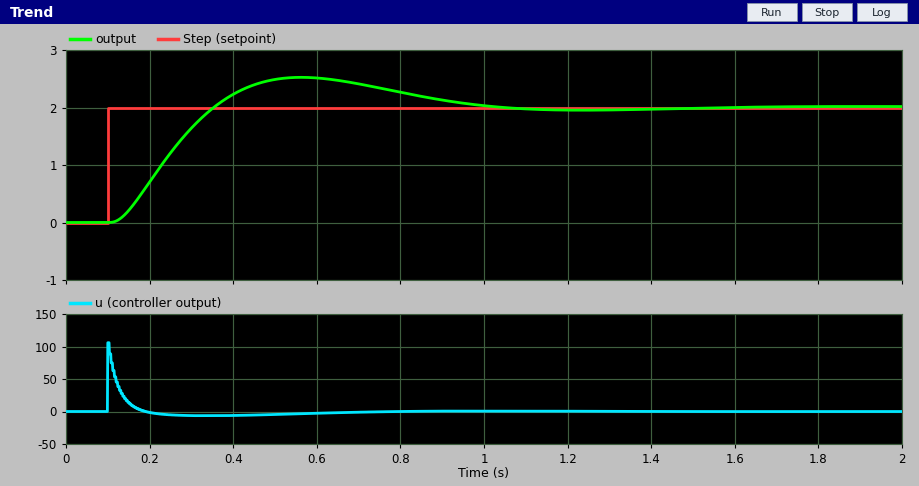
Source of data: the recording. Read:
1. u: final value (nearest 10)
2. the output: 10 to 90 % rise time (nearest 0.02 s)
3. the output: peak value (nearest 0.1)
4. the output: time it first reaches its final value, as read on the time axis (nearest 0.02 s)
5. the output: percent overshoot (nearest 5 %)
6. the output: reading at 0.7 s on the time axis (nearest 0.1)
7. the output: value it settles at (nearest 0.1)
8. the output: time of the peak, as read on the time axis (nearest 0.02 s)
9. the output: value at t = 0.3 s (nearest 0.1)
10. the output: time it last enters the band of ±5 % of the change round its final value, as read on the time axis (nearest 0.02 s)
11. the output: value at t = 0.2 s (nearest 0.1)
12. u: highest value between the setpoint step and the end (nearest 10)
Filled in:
0
0.18 s
2.5
0.36 s
25 %
2.4
2.0
0.56 s
1.6
0.92 s
0.7
110
